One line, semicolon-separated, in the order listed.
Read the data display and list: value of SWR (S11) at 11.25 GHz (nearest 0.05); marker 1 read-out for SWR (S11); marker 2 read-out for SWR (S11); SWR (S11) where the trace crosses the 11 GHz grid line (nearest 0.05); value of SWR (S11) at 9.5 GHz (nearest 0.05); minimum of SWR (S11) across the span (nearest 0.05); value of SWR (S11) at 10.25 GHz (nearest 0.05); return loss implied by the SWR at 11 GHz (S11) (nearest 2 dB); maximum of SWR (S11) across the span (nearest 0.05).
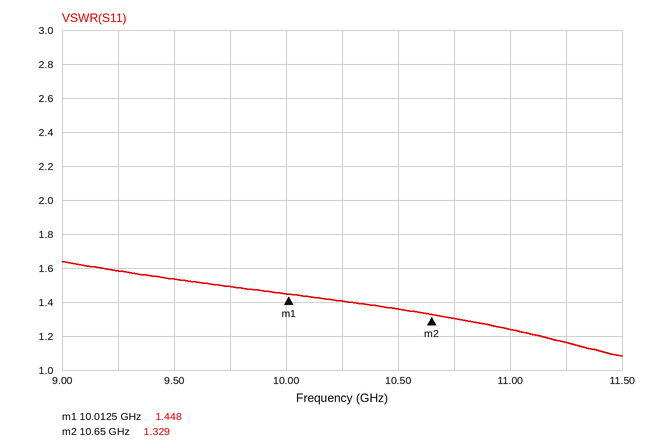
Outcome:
1.15; 1.448; 1.329; 1.25; 1.55; 1.10; 1.40; 20 dB; 1.65
